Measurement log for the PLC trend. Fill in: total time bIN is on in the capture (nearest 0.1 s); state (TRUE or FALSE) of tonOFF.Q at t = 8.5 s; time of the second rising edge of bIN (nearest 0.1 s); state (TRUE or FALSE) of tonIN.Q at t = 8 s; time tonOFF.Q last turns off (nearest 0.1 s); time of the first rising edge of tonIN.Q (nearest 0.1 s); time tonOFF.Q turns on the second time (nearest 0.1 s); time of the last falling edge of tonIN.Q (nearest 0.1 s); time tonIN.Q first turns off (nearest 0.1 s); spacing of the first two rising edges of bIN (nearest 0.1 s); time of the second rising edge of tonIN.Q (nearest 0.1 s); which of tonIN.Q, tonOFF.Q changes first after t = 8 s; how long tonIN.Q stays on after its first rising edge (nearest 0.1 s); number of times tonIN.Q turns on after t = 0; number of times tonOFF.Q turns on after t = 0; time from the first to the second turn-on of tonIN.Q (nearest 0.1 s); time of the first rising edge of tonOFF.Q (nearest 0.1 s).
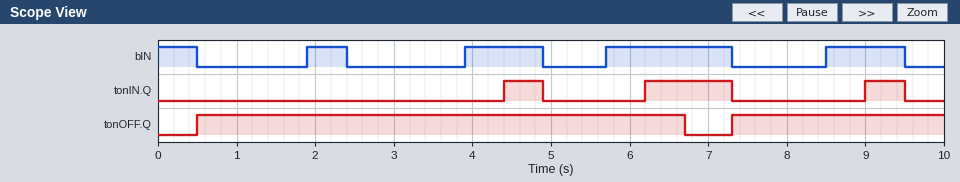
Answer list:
4.6 s
TRUE
3.9 s
FALSE
6.7 s
4.4 s
7.3 s
9.5 s
4.9 s
2.0 s
6.2 s
tonIN.Q
0.5 s
3
2
1.8 s
0.5 s
